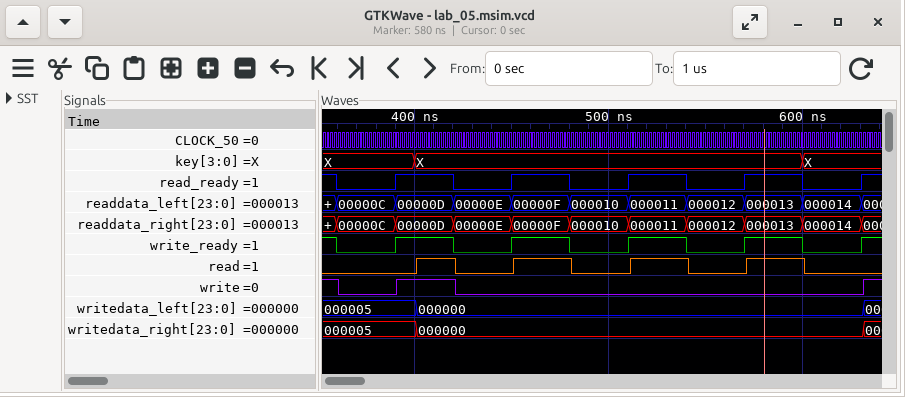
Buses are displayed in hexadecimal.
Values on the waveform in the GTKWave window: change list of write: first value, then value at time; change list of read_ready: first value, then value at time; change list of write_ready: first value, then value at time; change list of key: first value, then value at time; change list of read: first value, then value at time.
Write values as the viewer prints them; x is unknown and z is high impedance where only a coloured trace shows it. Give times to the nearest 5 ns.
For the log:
1, 0 at 360 ns, 1 at 390 ns, 0 at 420 ns, 1 at 630 ns
1, 0 at 360 ns, 1 at 390 ns, 0 at 420 ns, 1 at 450 ns, 0 at 480 ns, 1 at 510 ns, 0 at 540 ns, 1 at 570 ns, 0 at 600 ns, 1 at 630 ns
1, 0 at 360 ns, 1 at 390 ns, 0 at 420 ns, 1 at 450 ns, 0 at 480 ns, 1 at 510 ns, 0 at 540 ns, 1 at 570 ns, 0 at 600 ns, 1 at 630 ns
X, X at 400 ns, X at 600 ns
0, 1 at 400 ns, 0 at 420 ns, 1 at 450 ns, 0 at 480 ns, 1 at 510 ns, 0 at 540 ns, 1 at 570 ns, 0 at 600 ns
